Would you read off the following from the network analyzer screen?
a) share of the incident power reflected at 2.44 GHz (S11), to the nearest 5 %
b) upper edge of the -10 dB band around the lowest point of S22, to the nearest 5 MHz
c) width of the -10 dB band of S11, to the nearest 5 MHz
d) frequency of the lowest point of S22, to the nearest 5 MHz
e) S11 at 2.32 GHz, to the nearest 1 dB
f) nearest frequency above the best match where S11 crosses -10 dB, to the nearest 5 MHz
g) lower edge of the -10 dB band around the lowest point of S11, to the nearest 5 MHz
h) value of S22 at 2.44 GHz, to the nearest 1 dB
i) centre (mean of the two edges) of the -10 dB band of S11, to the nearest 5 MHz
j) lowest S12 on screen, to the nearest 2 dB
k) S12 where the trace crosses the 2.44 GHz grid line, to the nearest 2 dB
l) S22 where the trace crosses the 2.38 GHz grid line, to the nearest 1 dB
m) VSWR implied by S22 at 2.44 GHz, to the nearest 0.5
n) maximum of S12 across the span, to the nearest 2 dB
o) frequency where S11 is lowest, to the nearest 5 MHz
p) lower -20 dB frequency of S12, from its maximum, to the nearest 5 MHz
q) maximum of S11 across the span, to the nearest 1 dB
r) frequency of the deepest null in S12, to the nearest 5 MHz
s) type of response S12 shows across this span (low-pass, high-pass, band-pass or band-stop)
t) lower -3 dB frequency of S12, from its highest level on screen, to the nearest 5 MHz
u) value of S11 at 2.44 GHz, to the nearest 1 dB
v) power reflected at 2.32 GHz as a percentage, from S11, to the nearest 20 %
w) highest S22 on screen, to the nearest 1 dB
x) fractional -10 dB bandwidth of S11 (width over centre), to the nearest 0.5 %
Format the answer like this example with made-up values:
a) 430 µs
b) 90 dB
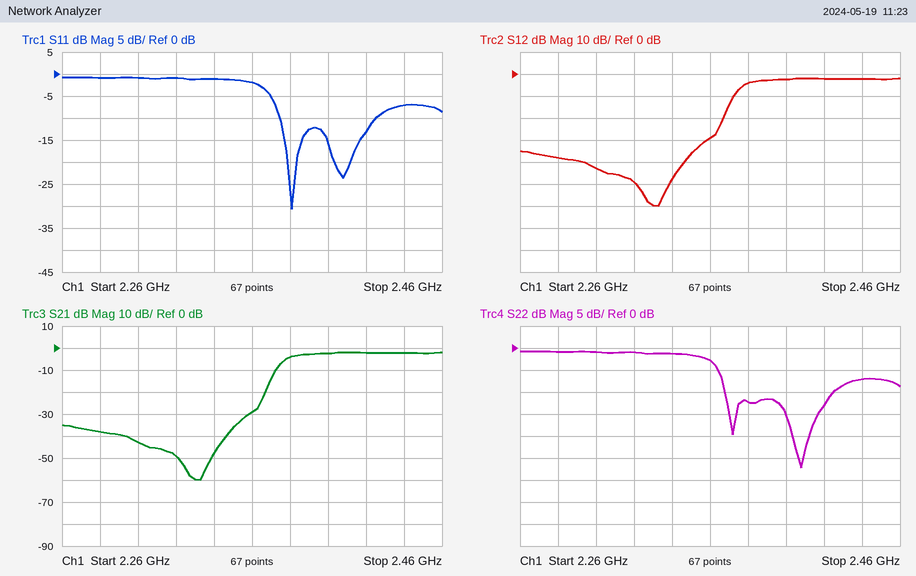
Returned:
a) 20 %
b) 2.425 GHz
c) 50 MHz
d) 2.410 GHz
e) -1 dB
f) 2.425 GHz
g) 2.375 GHz
h) -7 dB
i) 2.400 GHz
j) -60 dB
k) -2 dB
l) -12 dB
m) 2.5
n) -2 dB
o) 2.380 GHz
p) 2.365 GHz
q) -1 dB
r) 2.335 GHz
s) high-pass
t) 2.380 GHz
u) -7 dB
v) 80 %
w) -1 dB
x) 2.0 %
